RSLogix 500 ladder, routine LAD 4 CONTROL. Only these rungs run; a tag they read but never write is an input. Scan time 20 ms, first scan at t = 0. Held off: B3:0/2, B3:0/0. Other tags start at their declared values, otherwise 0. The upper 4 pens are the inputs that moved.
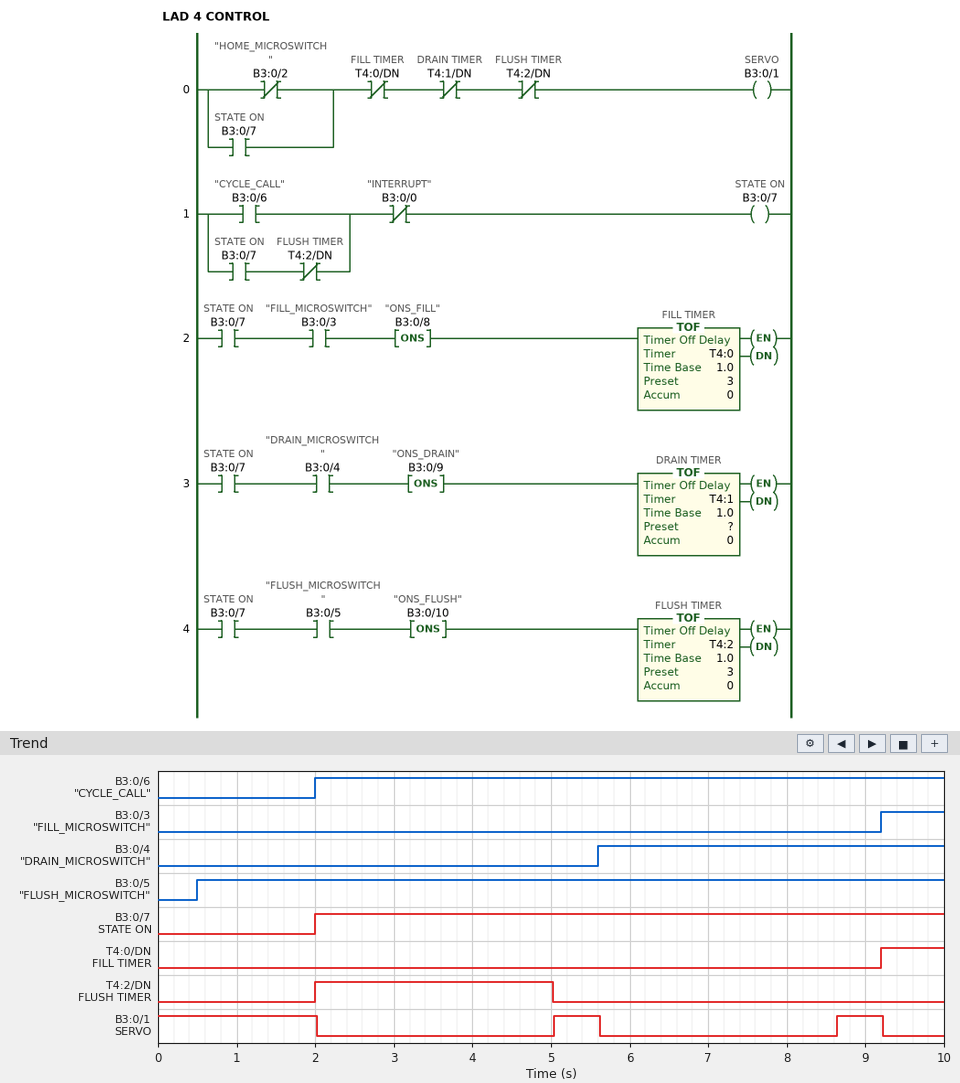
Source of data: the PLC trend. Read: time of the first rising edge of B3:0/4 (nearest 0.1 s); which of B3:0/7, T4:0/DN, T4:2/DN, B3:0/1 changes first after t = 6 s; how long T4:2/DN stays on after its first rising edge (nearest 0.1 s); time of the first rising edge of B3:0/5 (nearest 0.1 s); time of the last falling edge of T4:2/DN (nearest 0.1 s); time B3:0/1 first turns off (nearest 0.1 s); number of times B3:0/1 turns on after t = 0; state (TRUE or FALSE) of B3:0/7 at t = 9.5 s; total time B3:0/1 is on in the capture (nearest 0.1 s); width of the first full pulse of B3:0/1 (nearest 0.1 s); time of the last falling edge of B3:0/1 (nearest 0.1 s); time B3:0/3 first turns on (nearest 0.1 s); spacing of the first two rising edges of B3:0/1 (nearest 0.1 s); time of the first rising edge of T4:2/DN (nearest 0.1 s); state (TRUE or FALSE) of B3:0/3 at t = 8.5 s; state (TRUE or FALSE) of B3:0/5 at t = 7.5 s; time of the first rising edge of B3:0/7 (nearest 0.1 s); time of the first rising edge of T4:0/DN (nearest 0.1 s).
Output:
5.6 s
B3:0/1
3.0 s
0.5 s
5.0 s
2.0 s
2
TRUE
3.2 s
0.6 s
9.2 s
9.2 s
3.6 s
2.0 s
FALSE
TRUE
2.0 s
9.2 s
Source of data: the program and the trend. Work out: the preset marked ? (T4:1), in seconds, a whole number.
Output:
3 s
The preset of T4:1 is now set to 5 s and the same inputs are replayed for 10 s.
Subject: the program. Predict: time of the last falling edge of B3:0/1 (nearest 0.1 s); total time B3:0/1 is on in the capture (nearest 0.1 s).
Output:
5.6 s
2.6 s
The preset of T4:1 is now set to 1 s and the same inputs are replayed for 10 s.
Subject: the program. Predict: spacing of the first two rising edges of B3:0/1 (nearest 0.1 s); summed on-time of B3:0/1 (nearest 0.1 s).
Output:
1.6 s
5.2 s
